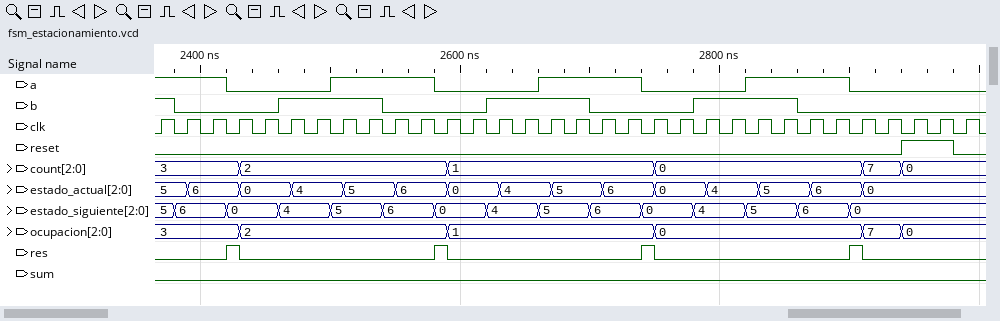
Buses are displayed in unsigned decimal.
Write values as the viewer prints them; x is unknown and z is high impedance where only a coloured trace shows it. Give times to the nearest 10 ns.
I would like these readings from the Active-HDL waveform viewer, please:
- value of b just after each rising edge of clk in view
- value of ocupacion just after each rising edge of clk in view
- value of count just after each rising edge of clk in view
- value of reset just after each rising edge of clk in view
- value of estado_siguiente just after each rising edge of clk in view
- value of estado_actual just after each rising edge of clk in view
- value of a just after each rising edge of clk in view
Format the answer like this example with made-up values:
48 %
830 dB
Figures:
1 0 0 0 0 1 1 1 1 0 0 0 0 1 1 1 1 0 0 0 0 1 1 1 1 0 0 0 0 0 0 0
3, 3, 3, 2, 2, 2, 2, 2, 2, 2, 2, 1, 1, 1, 1, 1, 1, 1, 1, 0, 0, 0, 0, 0, 0, 0, 0, 7, 7, 0, 0, 0
3, 3, 3, 2, 2, 2, 2, 2, 2, 2, 2, 1, 1, 1, 1, 1, 1, 1, 1, 0, 0, 0, 0, 0, 0, 0, 0, 7, 7, 0, 0, 0
0 0 0 0 0 0 0 0 0 0 0 0 0 0 0 0 0 0 0 0 0 0 0 0 0 0 0 0 0 1 1 0
5, 6, 6, 0, 0, 4, 4, 5, 5, 6, 6, 0, 0, 4, 4, 5, 5, 6, 6, 0, 0, 4, 4, 5, 5, 6, 6, 0, 0, 0, 0, 0
5, 6, 6, 0, 0, 4, 4, 5, 5, 6, 6, 0, 0, 4, 4, 5, 5, 6, 6, 0, 0, 4, 4, 5, 5, 6, 6, 0, 0, 0, 0, 0
1 1 1 0 0 0 0 1 1 1 1 0 0 0 0 1 1 1 1 0 0 0 0 1 1 1 1 0 0 0 0 0
